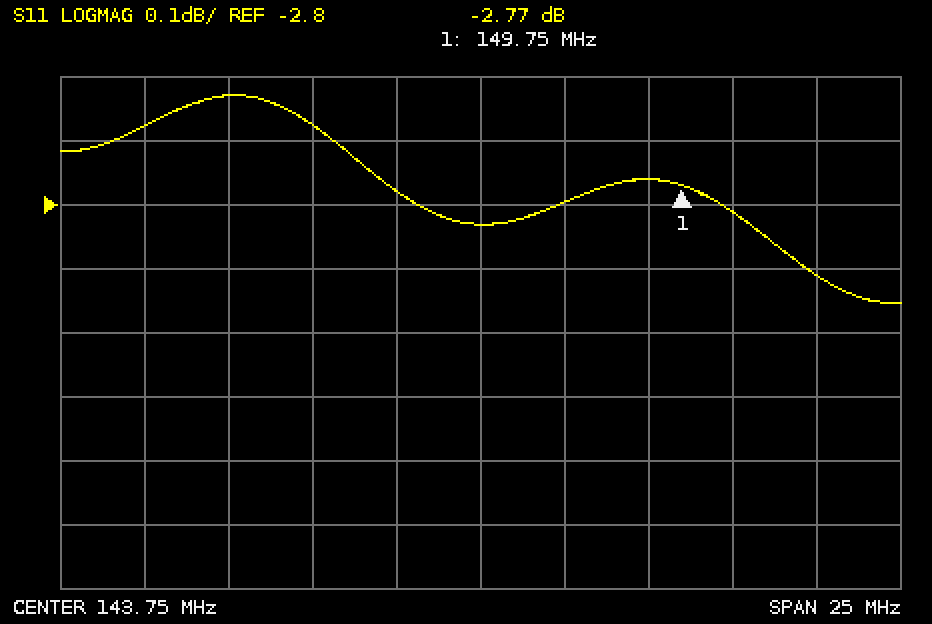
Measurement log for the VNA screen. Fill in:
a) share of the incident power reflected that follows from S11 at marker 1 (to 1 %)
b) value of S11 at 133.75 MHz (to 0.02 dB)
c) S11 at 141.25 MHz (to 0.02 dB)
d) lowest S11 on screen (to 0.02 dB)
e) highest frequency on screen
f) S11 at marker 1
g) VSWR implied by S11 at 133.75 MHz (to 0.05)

53 %
-2.68 dB
-2.78 dB
-2.96 dB
156.25 MHz
-2.77 dB
6.55
